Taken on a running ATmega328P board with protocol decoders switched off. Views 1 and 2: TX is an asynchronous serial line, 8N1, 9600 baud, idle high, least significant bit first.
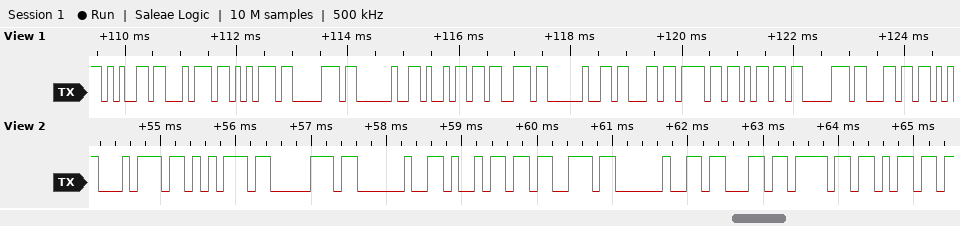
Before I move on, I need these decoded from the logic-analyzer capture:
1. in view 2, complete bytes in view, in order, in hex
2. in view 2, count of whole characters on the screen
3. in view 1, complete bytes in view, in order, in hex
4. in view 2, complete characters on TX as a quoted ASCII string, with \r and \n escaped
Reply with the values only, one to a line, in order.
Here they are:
74 75 70 20 69 73 20 63 6F 6D
10
0x65 0x74 0x75 0x70 0x20 0x69 0x73 0x20 0x63 0x6F 0x6D 0x70 0x6C
"tup is com"
